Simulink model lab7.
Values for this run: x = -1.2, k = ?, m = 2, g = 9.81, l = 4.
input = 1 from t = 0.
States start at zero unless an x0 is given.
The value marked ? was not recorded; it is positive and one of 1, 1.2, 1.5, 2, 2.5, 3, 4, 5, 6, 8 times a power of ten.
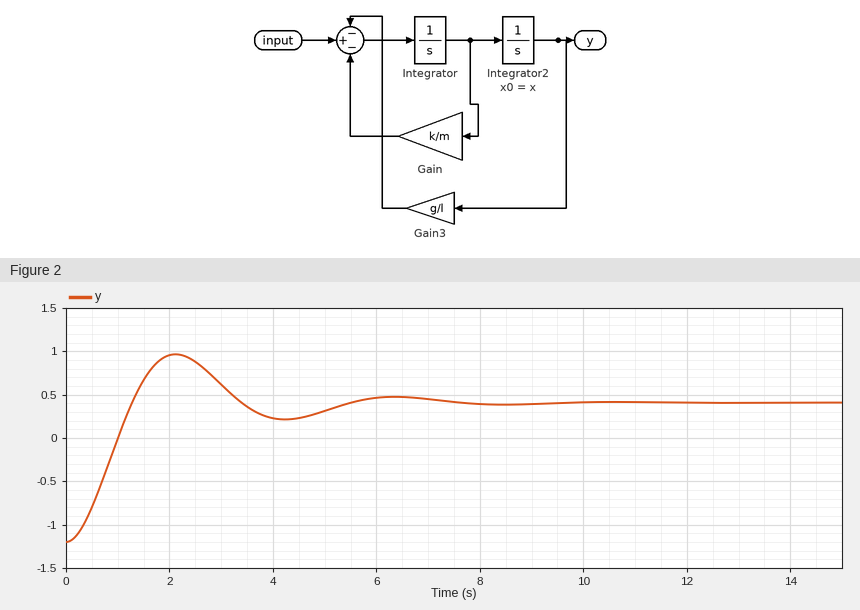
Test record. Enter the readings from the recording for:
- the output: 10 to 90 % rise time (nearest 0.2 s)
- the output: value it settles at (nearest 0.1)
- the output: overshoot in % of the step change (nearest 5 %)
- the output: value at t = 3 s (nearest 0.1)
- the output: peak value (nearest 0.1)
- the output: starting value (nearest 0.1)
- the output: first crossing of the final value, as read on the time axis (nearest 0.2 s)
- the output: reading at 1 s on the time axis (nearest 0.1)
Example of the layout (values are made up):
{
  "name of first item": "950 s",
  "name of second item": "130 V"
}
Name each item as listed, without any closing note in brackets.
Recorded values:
{
  "the output: 10 to 90 % rise time": "0.8 s",
  "the output: value it settles at": "0.4",
  "the output: overshoot in % of the step change": "35 %",
  "the output: value at t = 3 s": "0.6",
  "the output: peak value": "1.0",
  "the output: starting value": "-1.2",
  "the output: first crossing of the final value, as read on the time axis": "1.2 s",
  "the output: reading at 1 s on the time axis": "0.0"
}
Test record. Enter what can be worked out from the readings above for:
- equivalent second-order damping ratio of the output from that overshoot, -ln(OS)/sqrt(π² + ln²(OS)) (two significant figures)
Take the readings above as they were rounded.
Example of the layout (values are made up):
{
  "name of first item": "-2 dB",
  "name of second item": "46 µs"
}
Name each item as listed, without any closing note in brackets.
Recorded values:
{
  "equivalent second-order damping ratio of the output from that overshoot, -ln(OS)/sqrt(π² + ln²(OS))": "0.32"
}
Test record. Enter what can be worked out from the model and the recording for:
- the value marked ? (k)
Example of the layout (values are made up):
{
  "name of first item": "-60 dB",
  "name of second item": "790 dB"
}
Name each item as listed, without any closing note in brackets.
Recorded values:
{
  "the value marked ?": "2"
}
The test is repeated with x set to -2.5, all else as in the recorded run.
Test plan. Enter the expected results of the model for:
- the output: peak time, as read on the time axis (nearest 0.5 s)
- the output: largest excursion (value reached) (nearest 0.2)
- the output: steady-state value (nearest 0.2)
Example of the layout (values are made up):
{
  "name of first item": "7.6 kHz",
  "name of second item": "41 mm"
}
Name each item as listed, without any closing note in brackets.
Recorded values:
{
  "the output: peak time, as read on the time axis": "2.0 s",
  "the output: largest excursion (value reached)": "1.4",
  "the output: steady-state value": "0.4"
}
